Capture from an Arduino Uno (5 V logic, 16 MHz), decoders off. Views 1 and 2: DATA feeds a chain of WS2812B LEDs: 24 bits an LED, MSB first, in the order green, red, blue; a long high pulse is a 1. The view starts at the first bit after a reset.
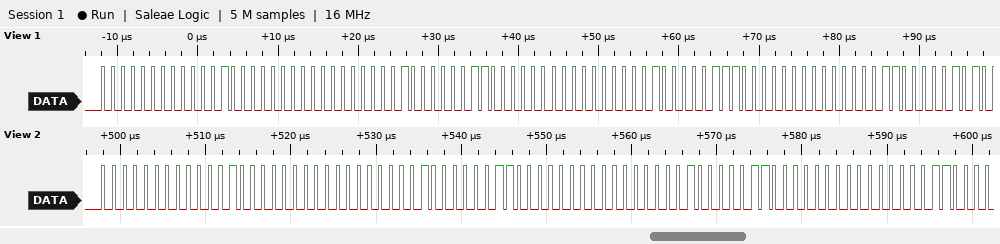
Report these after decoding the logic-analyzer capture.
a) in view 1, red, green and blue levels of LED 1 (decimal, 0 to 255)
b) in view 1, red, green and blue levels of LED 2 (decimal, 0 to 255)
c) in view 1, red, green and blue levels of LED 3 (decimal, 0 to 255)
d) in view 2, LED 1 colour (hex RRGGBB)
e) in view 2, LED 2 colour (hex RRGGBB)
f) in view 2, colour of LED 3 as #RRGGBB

8, 0, 0
6, 2, 0
7, 1, 0
#080000
#060200
#060100
